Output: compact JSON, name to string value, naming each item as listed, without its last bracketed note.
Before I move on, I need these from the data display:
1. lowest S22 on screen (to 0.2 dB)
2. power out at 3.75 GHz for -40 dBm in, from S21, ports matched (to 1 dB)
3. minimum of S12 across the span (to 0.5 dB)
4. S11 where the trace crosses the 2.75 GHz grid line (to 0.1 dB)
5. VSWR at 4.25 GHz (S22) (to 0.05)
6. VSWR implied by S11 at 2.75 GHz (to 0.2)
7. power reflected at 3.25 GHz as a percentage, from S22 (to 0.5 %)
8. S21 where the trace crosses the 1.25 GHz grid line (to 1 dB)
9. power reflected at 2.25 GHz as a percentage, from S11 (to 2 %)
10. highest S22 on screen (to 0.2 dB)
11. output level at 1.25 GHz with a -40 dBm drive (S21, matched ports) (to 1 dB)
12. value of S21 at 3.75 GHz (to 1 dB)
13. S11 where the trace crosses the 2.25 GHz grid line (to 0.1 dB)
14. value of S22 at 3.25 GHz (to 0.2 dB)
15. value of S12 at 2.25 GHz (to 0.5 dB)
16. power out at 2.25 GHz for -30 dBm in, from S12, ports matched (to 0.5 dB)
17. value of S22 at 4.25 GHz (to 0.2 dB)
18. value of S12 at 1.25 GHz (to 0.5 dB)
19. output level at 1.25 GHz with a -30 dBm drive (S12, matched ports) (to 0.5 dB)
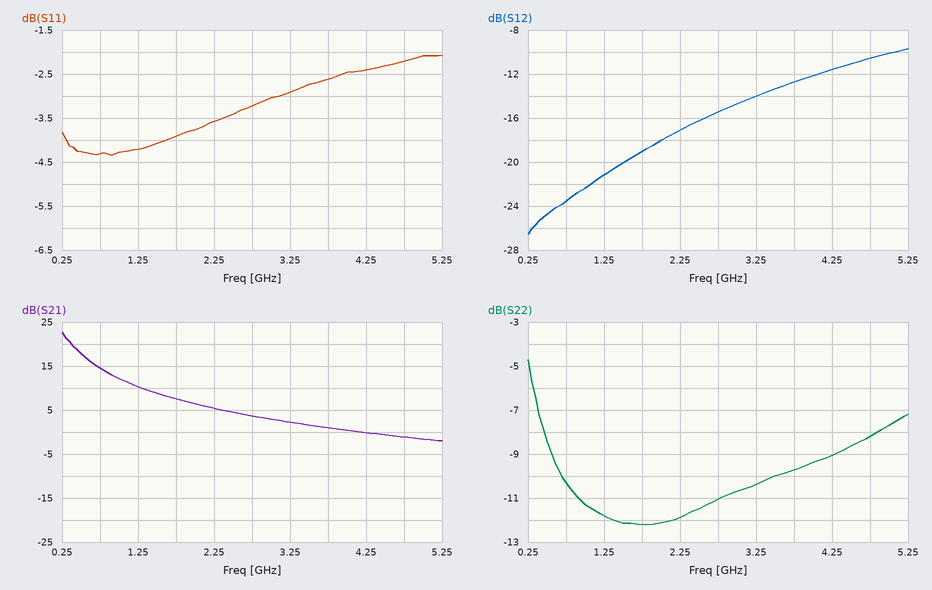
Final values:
{"lowest S22 on screen": "-12.2 dB", "power out at 3.75 GHz for -40 dBm in, from S21, ports matched": "-39 dBm", "minimum of S12 across the span": "-26.5 dB", "S11 where the trace crosses the 2.75 GHz grid line": "-3.2 dB", "VSWR at 4.25 GHz (S22)": "2.10", "VSWR implied by S11 at 2.75 GHz": "5.4", "power reflected at 3.25 GHz as a percentage, from S22": "9.0 %", "S21 where the trace crosses the 1.25 GHz grid line": "10 dB", "power reflected at 2.25 GHz as a percentage, from S11": "44 %", "highest S22 on screen": "-4.8 dB", "output level at 1.25 GHz with a -40 dBm drive (S21, matched ports)": "-30 dBm", "value of S21 at 3.75 GHz": "1 dB", "S11 where the trace crosses the 2.25 GHz grid line": "-3.6 dB", "value of S22 at 3.25 GHz": "-10.4 dB", "value of S12 at 2.25 GHz": "-17.0 dB", "power out at 2.25 GHz for -30 dBm in, from S12, ports matched": "-47.0 dBm", "value of S22 at 4.25 GHz": "-9.0 dB", "value of S12 at 1.25 GHz": "-21.0 dB", "output level at 1.25 GHz with a -30 dBm drive (S12, matched ports)": "-51.0 dBm"}
